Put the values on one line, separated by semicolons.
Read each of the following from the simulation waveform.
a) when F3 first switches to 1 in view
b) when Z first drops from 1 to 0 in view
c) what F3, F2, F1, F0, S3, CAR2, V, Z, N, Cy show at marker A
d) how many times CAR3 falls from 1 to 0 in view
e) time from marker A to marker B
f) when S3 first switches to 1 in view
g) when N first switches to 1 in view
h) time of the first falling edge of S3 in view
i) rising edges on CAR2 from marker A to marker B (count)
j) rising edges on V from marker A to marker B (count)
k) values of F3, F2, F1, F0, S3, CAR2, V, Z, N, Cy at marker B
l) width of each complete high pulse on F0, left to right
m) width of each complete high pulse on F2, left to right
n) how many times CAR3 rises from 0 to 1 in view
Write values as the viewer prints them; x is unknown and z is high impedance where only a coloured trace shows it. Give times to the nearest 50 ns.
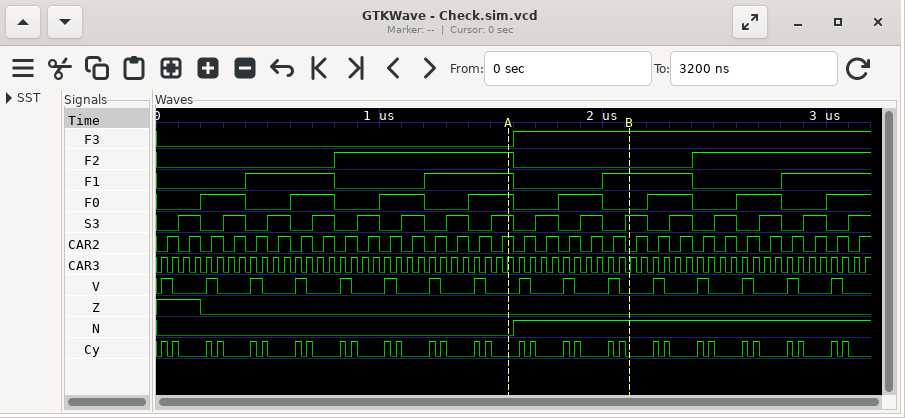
1600 ns; 200 ns; F3=0, F2=1, F1=1, F0=1, S3=1, CAR2=1, V=0, Z=0, N=0, Cy=0; 63; 550 ns; 100 ns; 1600 ns; 200 ns; 5; 3; F3=1, F2=0, F1=1, F0=0, S3=1, CAR2=0, V=0, Z=0, N=1, Cy=0; 200 ns, 200 ns, 200 ns, 200 ns, 200 ns, 200 ns, 200 ns; 800 ns; 64
